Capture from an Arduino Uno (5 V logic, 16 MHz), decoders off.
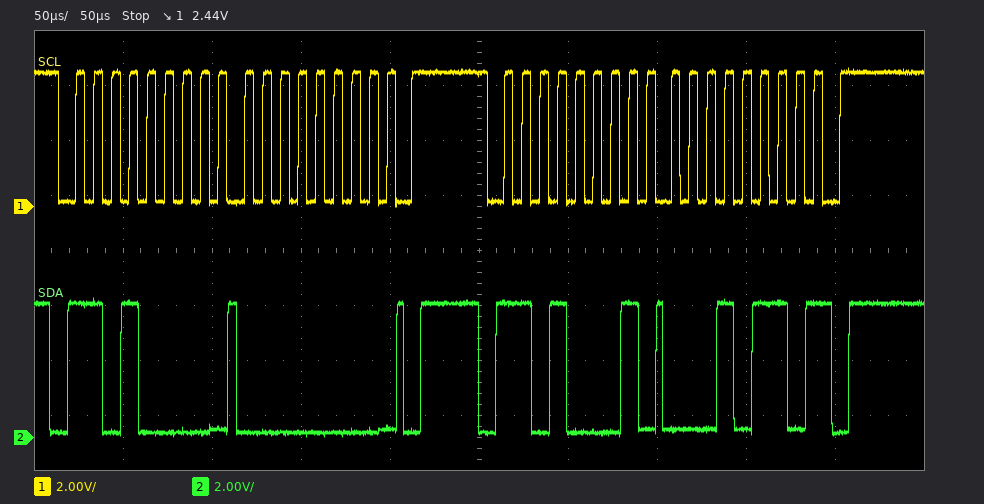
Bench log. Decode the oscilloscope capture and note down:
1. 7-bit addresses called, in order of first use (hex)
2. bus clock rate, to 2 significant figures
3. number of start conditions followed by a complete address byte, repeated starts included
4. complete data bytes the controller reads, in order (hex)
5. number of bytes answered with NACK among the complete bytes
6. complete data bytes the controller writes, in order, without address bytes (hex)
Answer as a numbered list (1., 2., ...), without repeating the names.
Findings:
1. 0x68
2. 100 kHz
3. 2
4. 16
5. 1
6. 00
